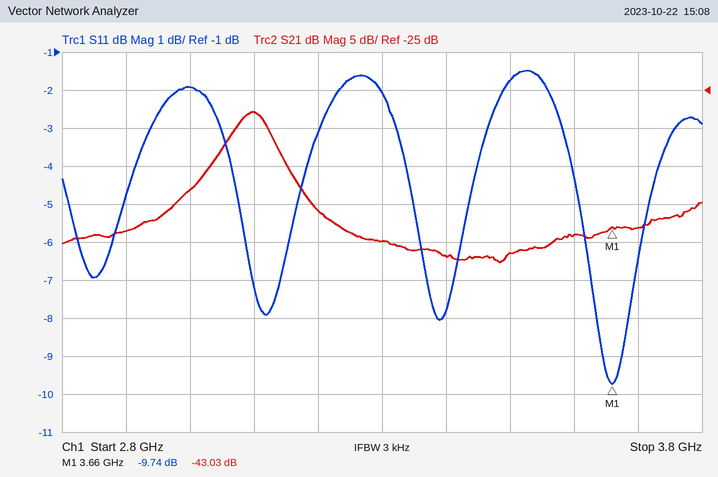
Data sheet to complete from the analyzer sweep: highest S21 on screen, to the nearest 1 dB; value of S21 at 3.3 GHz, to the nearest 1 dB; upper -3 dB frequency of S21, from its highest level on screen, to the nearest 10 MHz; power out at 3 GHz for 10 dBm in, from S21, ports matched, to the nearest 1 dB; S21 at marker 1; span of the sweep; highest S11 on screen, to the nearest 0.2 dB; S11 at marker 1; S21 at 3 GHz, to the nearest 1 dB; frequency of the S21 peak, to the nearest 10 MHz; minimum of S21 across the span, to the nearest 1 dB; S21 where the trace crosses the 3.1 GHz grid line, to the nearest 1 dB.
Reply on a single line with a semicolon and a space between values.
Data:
-28 dB; -45 dB; 3.13 GHz; -28 dBm; -43.03 dB; 1 GHz; -1.4 dB; -9.74 dB; -38 dB; 3.10 GHz; -48 dB; -28 dB
